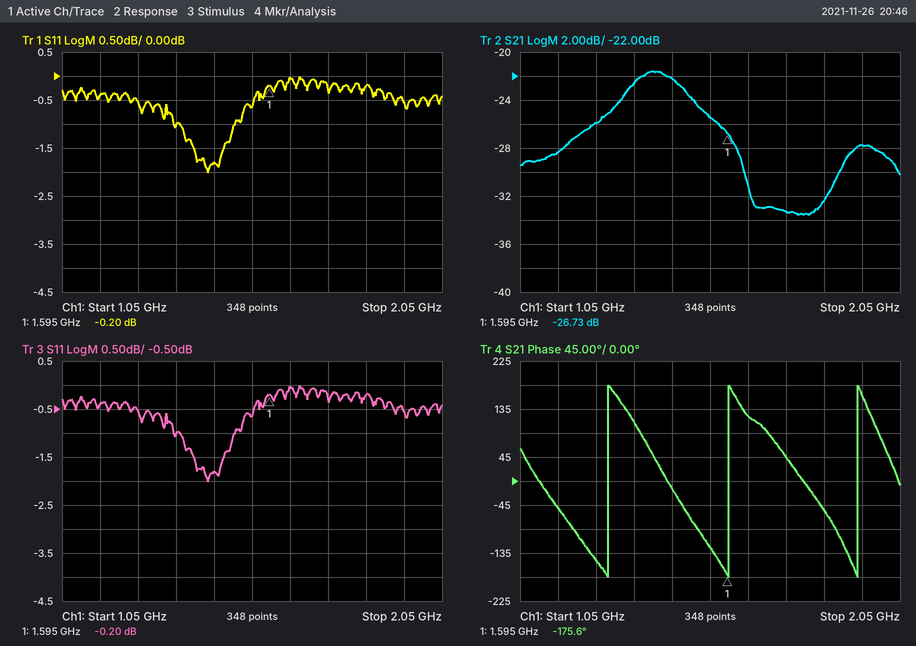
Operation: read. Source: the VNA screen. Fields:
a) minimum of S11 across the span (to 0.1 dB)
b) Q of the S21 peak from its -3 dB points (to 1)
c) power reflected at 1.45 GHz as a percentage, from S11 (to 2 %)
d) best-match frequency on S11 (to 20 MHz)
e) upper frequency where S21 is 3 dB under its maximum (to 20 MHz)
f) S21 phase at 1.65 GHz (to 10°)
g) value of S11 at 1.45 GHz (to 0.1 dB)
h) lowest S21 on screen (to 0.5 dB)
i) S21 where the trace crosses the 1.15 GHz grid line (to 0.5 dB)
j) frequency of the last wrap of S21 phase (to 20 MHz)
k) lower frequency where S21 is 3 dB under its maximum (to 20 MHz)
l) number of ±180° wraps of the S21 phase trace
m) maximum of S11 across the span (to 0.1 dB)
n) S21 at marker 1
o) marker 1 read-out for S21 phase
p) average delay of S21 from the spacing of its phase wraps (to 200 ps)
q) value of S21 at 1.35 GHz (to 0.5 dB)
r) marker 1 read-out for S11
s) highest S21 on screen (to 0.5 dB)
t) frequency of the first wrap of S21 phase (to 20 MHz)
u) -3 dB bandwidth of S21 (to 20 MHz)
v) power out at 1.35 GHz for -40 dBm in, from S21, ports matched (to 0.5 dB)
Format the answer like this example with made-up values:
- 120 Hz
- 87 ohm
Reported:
- -2.0 dB
- 6
- 66 %
- 1.44 GHz
- 1.52 GHz
- 120°
- -1.8 dB
- -33.5 dB
- -28.5 dB
- 1.94 GHz
- 1.30 GHz
- 3
- 0.0 dB
- -26.73 dB
- -175.6°
- 3.0 ns
- -22.5 dB
- -0.20 dB
- -21.5 dB
- 1.28 GHz
- 220 MHz
- -62.5 dBm
